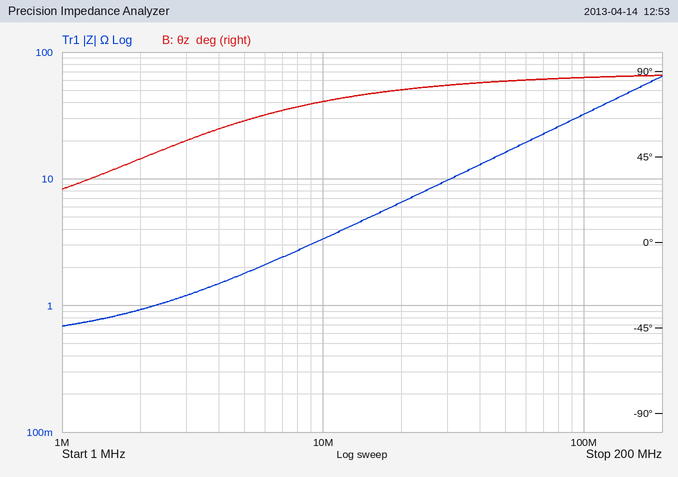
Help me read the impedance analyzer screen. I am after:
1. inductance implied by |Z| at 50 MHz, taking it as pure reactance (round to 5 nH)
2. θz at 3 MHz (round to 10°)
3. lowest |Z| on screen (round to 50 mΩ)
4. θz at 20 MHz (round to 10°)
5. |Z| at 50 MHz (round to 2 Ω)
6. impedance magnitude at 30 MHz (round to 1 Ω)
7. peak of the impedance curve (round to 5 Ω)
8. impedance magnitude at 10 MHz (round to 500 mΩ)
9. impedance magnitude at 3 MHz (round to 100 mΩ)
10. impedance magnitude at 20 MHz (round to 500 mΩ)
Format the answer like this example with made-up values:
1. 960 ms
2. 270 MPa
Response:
1. 50 nH
2. 50°
3. 700 mΩ
4. 80°
5. 16 Ω
6. 10 Ω
7. 65 Ω
8. 3.5 Ω
9. 1.2 Ω
10. 6.5 Ω
